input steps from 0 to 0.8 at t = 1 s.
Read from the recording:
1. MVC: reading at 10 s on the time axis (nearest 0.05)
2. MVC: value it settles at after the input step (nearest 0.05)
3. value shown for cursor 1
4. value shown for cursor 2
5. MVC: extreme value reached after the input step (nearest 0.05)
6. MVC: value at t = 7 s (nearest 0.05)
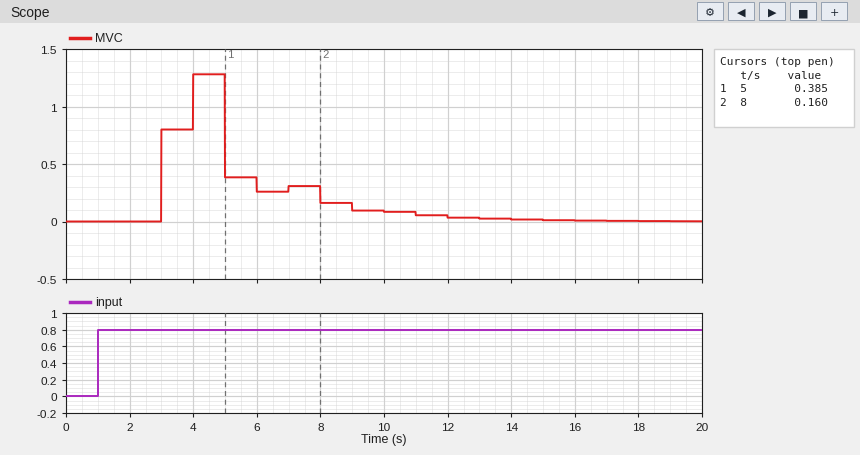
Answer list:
0.10
0.00
0.385
0.160
1.30
0.30
